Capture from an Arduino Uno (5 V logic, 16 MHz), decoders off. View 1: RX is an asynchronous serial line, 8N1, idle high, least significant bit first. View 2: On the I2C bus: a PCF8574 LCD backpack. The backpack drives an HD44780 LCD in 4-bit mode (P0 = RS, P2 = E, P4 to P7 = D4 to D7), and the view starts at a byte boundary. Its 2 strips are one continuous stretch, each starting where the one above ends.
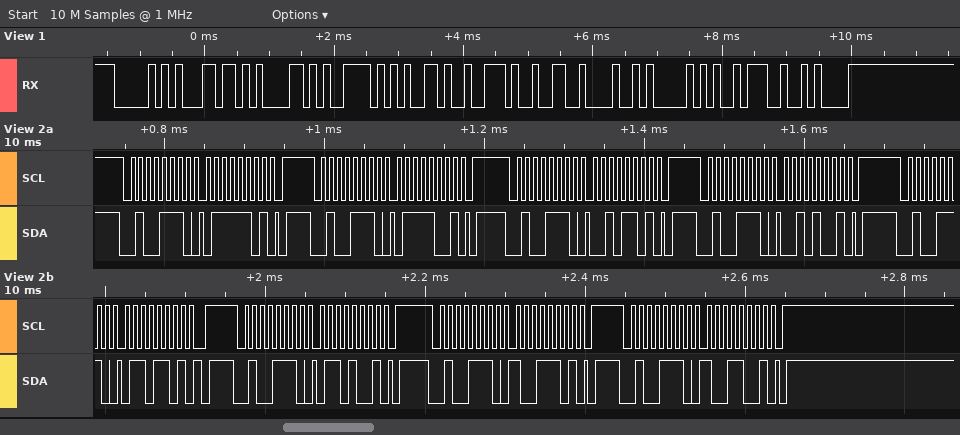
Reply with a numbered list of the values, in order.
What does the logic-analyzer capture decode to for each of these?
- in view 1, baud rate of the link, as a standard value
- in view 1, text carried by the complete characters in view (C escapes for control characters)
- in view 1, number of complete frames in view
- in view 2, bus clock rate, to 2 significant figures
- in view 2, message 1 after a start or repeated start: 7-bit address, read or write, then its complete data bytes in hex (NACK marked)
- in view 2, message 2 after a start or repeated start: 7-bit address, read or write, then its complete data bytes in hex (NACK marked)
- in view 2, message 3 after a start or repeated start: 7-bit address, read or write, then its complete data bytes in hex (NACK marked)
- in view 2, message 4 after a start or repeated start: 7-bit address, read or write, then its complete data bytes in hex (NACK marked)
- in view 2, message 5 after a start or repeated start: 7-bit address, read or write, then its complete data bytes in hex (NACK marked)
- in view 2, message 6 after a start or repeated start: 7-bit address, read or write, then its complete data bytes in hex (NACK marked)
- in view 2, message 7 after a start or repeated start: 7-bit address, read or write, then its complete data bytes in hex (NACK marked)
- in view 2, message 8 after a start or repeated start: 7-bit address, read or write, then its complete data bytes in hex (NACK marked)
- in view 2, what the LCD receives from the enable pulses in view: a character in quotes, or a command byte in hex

1. 9600 baud
2. "Player2HP:\n"
3. 11
4. 100 kHz
5. 0x27 write: 7D
6. 0x27 write: 79
7. 0x27 write: 2D
8. 0x27 write: 29
9. 0x27 write: 6D
10. 0x27 write: 69
11. 0x27 write: 9D
12. 0x27 write: 99
13. 'r' 'i'
